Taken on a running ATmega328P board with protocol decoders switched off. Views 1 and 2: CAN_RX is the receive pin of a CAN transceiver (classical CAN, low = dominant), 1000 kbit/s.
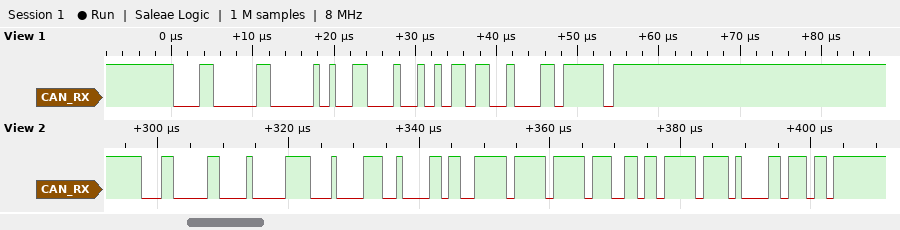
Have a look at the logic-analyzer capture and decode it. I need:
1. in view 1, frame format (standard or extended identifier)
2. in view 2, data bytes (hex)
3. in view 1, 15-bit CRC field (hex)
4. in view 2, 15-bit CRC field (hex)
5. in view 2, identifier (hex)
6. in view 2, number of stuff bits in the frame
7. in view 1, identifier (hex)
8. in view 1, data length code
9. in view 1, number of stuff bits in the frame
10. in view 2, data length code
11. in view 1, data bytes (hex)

standard
38 87 21 B3 FF FF 36 FF
0x646F
0x50DD
0x182
6
0x182
2
2
8
62 56
